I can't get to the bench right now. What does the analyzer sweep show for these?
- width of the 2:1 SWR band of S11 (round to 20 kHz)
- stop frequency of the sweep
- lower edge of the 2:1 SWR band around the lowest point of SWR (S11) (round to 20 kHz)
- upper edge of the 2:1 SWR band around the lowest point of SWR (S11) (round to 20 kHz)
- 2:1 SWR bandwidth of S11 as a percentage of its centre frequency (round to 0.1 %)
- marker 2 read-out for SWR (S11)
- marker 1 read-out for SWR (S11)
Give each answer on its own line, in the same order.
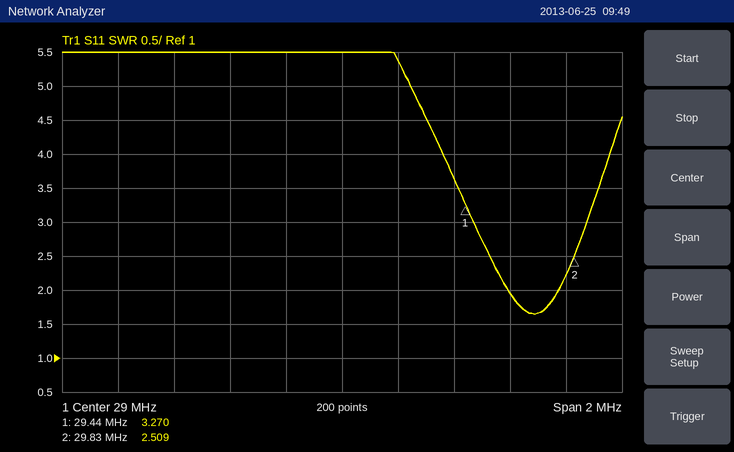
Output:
180 kHz
30 MHz
29.60 MHz
29.78 MHz
0.6 %
2.509
3.270
